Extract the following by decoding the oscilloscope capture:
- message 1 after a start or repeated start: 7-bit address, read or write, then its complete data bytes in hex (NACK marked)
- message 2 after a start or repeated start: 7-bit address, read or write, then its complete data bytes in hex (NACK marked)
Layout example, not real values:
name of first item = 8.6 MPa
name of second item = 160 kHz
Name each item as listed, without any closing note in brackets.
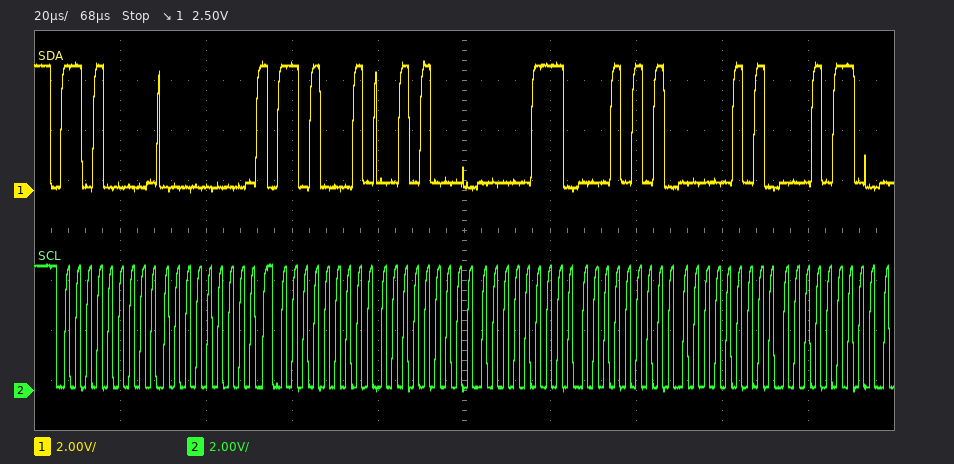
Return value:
message 1 after a start or repeated start: 7-bit address, read or write, then its complete data bytes in hex = 0x68 write: 00
message 2 after a start or repeated start: 7-bit address, read or write, then its complete data bytes in hex = 0x68 read: 28 07 15 05 16
